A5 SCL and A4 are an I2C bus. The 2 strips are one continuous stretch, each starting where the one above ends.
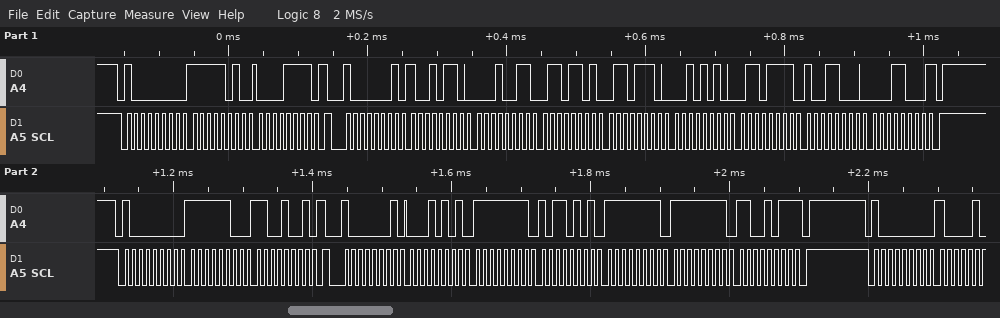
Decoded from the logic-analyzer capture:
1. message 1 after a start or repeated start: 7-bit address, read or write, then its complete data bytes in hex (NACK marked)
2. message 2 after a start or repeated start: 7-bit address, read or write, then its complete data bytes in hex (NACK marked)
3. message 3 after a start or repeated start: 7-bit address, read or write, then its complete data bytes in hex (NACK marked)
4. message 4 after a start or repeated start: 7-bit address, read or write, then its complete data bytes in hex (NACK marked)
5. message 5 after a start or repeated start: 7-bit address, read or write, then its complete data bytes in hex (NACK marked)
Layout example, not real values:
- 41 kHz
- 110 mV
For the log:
- 0x40 write: FA 0F
- 0x40 read: 96 13 6D 6E 2A 6F 98 18 NACK
- 0x40 write: FC C9
- 0x40 read: 15 FF B5 FF FF CB NACK
- 0x40 write
